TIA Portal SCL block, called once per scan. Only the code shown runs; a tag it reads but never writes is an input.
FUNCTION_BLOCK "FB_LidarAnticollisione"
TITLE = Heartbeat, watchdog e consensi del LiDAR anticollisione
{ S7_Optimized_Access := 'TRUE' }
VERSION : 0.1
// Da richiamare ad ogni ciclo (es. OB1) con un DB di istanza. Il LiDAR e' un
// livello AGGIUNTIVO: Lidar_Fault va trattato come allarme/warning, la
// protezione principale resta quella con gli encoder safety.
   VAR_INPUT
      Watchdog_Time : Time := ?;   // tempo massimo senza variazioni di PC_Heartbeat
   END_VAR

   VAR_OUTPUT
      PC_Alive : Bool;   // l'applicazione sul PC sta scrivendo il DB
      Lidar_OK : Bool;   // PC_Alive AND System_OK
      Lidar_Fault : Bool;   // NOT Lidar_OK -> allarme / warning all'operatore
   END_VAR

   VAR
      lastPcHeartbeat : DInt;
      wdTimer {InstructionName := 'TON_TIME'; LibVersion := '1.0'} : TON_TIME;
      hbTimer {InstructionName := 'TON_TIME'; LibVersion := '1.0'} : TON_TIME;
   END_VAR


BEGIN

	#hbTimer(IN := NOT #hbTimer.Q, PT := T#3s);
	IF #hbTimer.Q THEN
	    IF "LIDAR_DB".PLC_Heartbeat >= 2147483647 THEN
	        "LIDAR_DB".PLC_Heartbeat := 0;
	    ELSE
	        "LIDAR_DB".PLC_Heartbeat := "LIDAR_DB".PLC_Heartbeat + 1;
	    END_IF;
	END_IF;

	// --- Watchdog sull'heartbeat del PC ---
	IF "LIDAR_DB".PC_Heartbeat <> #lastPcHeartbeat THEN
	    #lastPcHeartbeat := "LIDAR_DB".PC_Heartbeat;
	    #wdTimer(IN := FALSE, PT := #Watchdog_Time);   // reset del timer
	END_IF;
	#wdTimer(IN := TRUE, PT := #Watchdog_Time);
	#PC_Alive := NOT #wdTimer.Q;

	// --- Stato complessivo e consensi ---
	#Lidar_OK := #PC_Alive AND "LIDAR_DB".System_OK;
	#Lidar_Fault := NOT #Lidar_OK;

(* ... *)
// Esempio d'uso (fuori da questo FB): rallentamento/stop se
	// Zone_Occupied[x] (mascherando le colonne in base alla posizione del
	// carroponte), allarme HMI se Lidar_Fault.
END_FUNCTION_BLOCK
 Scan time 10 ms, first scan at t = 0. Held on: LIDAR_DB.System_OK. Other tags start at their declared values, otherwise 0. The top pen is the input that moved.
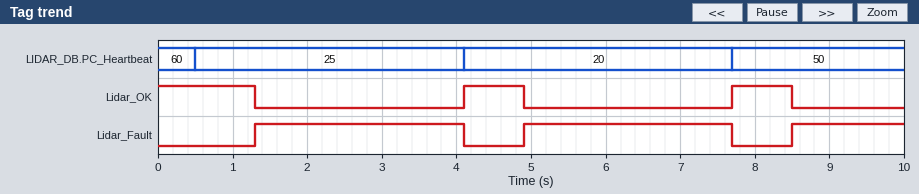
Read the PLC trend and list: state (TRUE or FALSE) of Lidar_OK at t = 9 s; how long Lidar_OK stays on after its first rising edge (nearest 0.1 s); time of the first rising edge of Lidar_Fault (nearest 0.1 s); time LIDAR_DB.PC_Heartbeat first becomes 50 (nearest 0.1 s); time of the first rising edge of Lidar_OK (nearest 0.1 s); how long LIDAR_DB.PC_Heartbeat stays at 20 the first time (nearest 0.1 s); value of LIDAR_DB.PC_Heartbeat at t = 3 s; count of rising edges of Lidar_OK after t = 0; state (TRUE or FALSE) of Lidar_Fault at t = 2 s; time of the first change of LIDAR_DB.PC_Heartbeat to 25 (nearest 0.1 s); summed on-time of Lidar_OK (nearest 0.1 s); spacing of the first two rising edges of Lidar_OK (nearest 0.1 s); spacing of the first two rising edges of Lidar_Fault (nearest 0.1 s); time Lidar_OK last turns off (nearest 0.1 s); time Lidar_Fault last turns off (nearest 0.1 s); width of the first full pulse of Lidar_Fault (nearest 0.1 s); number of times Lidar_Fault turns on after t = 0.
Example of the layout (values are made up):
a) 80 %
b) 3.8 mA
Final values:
a) FALSE
b) 0.8 s
c) 1.3 s
d) 7.7 s
e) 4.1 s
f) 3.6 s
g) 25
h) 2
i) TRUE
j) 0.5 s
k) 2.9 s
l) 3.6 s
m) 3.6 s
n) 8.5 s
o) 7.7 s
p) 2.8 s
q) 3
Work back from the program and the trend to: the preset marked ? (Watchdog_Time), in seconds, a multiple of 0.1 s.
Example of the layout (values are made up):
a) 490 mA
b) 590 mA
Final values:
a) 0.8 s
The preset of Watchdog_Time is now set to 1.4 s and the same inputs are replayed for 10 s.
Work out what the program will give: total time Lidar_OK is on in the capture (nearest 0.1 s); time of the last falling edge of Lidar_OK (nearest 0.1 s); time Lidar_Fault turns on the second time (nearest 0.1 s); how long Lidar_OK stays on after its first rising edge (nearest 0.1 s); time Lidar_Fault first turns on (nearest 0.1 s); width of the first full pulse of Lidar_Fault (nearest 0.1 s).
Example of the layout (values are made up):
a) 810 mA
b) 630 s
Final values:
a) 4.7 s
b) 9.1 s
c) 5.5 s
d) 1.4 s
e) 1.9 s
f) 2.2 s
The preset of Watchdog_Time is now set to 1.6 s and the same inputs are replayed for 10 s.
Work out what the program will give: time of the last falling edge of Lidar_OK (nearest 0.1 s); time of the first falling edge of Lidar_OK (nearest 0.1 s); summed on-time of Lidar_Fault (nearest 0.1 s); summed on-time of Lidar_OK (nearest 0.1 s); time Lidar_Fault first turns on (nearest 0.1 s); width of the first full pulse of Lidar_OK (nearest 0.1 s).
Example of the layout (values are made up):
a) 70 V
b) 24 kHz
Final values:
a) 9.3 s
b) 2.1 s
c) 4.7 s
d) 5.3 s
e) 2.1 s
f) 1.6 s
